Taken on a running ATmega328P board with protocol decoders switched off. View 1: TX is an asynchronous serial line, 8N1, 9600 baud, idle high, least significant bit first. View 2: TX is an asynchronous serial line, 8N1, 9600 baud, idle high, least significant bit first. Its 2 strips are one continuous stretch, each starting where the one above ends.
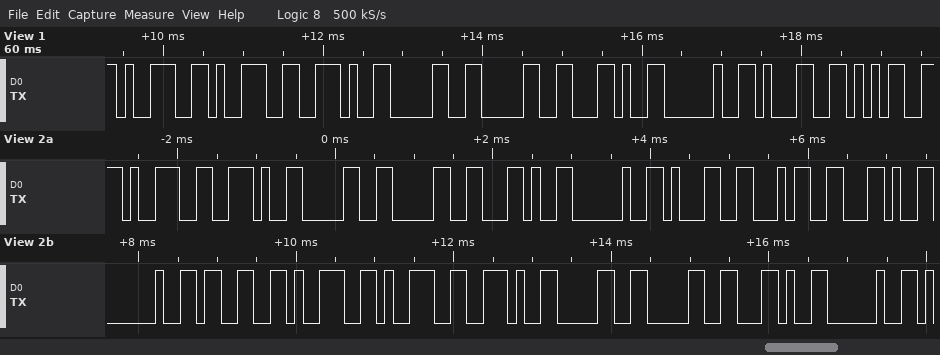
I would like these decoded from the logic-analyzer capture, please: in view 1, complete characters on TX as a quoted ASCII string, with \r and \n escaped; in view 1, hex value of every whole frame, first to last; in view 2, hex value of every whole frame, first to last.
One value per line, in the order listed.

"99.00, 15"
39 39 2E 30 30 2C 20 31 35
0x39 0x2E 0x30 0x30 0x2C 0x20 0x31 0x34 0x2C 0x20 0x33 0x39 0x39 0x2E 0x30 0x30 0x2C 0x20
